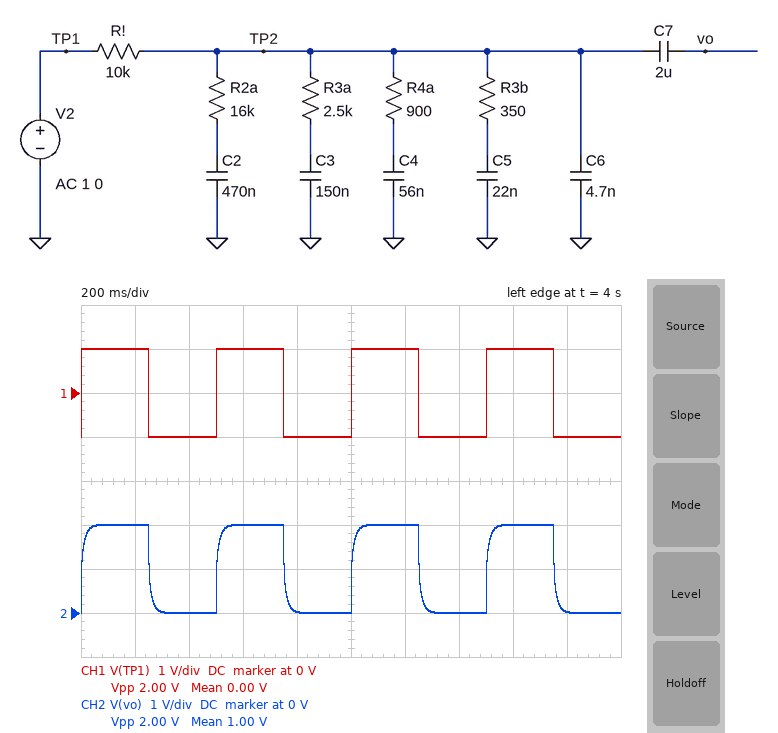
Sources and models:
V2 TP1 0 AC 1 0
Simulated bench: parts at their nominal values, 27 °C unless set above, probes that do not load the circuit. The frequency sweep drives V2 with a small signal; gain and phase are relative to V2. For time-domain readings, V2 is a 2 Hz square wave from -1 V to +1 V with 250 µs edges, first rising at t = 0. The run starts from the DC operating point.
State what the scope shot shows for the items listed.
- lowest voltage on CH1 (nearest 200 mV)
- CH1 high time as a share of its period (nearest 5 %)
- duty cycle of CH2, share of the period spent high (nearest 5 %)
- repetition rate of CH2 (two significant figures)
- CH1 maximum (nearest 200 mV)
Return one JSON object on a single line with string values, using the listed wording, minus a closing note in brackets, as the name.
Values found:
{"lowest voltage on CH1": "-1.0 V", "CH1 high time as a share of its period": "50 %", "duty cycle of CH2, share of the period spent high": "50 %", "repetition rate of CH2": "2.0 Hz", "CH1 maximum": "1.0 V"}
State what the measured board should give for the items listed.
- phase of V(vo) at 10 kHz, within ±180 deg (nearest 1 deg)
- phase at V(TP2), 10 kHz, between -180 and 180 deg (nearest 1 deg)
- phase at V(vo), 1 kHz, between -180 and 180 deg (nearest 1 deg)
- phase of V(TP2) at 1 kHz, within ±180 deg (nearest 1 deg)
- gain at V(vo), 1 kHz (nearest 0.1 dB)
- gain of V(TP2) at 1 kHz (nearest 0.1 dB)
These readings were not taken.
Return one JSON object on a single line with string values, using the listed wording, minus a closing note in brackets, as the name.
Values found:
{"phase of V(vo) at 10 kHz, within ±180 deg": "-40 deg", "phase at V(TP2), 10 kHz, between -180 and 180 deg": "-40 deg", "phase at V(vo), 1 kHz, between -180 and 180 deg": "-46 deg", "phase of V(TP2) at 1 kHz, within ±180 deg": "-46 deg", "gain at V(vo), 1 kHz": "-18.9 dB", "gain of V(TP2) at 1 kHz": "-18.9 dB"}
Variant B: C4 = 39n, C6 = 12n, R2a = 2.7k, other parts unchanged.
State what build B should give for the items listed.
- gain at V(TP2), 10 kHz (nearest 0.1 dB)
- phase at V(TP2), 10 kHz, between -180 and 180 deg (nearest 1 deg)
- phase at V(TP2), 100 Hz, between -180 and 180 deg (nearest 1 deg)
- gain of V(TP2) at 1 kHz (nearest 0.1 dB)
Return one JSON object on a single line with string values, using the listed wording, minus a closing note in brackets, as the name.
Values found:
{"gain at V(TP2), 10 kHz": "-30.3 dB", "phase at V(TP2), 10 kHz, between -180 and 180 deg": "-45 deg", "phase at V(TP2), 100 Hz, between -180 and 180 deg": "-50 deg", "gain of V(TP2) at 1 kHz": "-20.6 dB"}
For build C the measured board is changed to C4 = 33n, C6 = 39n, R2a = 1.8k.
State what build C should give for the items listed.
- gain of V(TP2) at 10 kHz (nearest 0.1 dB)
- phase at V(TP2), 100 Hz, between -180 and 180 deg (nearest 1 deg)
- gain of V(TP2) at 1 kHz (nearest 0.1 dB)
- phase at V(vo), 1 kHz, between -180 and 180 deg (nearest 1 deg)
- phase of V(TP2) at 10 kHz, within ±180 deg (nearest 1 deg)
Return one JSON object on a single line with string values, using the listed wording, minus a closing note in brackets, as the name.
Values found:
{"gain of V(TP2) at 10 kHz": "-33.5 dB", "phase at V(TP2), 100 Hz, between -180 and 180 deg": "-57 deg", "gain of V(TP2) at 1 kHz": "-22.4 dB", "phase at V(vo), 1 kHz, between -180 and 180 deg": "-39 deg", "phase of V(TP2) at 10 kHz, within ±180 deg": "-59 deg"}
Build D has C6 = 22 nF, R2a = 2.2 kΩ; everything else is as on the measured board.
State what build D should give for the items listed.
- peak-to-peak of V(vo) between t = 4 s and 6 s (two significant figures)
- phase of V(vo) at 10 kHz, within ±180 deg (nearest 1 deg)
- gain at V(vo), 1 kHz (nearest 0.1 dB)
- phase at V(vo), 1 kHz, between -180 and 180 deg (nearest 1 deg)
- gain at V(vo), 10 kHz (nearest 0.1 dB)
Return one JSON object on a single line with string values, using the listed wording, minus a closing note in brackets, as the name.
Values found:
{"peak-to-peak of V(vo) between t = 4 s and 6 s": "2.0 V", "phase of V(vo) at 10 kHz, within ±180 deg": "-49 deg", "gain at V(vo), 1 kHz": "-22.1 dB", "phase at V(vo), 1 kHz, between -180 and 180 deg": "-39 deg", "gain at V(vo), 10 kHz": "-31.6 dB"}
